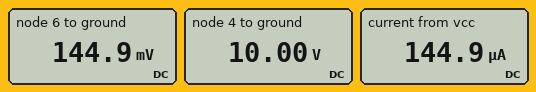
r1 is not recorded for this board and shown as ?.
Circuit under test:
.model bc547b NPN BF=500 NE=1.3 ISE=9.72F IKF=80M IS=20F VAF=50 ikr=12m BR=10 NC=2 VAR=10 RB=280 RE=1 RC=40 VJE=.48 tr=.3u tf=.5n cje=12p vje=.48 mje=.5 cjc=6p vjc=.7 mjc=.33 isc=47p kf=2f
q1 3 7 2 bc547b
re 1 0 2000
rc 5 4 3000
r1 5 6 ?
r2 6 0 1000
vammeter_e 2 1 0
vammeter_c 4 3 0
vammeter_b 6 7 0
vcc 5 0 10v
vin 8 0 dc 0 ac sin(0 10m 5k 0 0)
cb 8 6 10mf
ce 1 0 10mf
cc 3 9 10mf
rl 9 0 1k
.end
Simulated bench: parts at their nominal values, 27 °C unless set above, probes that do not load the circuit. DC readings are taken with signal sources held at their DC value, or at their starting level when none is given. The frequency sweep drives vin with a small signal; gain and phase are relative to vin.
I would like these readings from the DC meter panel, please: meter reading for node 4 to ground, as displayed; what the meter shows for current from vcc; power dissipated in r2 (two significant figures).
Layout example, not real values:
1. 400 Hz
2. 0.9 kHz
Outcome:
1. 10.00 V
2. 144.9 µA
3. 21 µW
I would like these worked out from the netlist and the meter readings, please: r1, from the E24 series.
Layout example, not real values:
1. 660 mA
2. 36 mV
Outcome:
1. 68 kΩ
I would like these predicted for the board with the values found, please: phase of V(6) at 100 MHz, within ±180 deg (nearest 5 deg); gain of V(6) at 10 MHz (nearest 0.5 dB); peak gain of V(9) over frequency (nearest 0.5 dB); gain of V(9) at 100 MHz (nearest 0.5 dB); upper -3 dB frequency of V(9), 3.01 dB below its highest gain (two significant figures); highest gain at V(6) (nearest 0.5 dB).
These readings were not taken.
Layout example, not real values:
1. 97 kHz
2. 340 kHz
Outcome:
1. 0 deg
2. 0 dB
3. -11.0 dB
4. -12.0 dB
5. 160 MHz
6. 0 dB
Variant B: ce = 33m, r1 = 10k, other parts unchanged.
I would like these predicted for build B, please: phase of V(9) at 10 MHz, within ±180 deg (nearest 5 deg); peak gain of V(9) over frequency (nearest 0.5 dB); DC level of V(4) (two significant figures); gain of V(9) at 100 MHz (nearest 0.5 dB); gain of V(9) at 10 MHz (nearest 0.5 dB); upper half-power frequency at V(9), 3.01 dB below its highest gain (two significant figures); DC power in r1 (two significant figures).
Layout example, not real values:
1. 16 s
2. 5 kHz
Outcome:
1. 135 deg
2. 13.0 dB
3. 9.5 V
4. -7.5 dB
5. 10.5 dB
6. 11 MHz
7. 8.3 mW
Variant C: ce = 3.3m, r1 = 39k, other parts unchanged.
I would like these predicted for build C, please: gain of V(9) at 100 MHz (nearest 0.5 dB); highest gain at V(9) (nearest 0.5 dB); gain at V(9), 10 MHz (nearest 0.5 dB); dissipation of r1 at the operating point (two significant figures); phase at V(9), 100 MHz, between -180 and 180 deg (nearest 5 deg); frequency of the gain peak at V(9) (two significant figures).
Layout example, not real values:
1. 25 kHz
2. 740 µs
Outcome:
1. -13.5 dB
2. -12.0 dB
3. -19.5 dB
4. 2.4 mW
5. -30 deg
6. 52 MHz
